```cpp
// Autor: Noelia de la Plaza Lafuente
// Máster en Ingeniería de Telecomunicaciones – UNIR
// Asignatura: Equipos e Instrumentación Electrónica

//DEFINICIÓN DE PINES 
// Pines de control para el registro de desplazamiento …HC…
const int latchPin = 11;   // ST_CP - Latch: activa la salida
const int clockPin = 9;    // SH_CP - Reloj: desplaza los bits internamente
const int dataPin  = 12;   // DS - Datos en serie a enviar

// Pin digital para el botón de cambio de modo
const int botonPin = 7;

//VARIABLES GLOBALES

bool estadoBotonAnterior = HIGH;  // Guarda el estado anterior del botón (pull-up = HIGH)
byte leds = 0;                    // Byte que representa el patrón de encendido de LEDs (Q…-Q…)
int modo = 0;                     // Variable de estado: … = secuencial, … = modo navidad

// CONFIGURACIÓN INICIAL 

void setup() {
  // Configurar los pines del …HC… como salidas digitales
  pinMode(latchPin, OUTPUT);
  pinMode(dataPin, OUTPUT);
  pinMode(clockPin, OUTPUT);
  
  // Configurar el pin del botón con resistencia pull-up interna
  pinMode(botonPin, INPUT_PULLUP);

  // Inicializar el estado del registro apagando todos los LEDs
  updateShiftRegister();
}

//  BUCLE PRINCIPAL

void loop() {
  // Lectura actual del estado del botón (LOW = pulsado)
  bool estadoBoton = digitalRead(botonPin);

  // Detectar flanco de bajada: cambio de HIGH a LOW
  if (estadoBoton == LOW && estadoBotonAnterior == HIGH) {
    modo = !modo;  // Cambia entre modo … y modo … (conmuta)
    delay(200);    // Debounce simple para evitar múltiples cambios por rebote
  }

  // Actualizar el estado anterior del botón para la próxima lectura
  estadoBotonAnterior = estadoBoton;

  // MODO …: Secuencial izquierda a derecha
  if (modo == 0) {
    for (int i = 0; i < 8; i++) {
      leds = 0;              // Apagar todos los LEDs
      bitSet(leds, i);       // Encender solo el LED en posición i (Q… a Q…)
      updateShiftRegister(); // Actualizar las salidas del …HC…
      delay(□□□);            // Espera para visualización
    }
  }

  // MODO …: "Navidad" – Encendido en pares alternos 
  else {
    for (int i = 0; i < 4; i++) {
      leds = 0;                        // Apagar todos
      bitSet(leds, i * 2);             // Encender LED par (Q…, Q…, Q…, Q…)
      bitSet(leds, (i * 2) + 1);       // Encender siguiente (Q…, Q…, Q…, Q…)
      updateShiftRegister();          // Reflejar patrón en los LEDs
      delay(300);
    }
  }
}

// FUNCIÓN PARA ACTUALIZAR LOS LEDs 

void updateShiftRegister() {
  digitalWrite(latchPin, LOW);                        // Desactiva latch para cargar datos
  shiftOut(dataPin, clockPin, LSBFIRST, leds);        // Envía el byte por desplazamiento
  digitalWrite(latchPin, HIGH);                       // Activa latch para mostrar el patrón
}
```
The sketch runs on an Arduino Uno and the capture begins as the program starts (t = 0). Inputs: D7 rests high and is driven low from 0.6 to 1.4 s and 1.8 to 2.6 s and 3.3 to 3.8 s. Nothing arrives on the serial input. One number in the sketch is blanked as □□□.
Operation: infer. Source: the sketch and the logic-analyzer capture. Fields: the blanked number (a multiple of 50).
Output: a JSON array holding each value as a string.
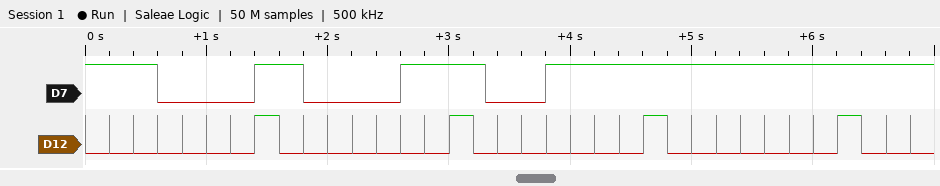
["200"]
